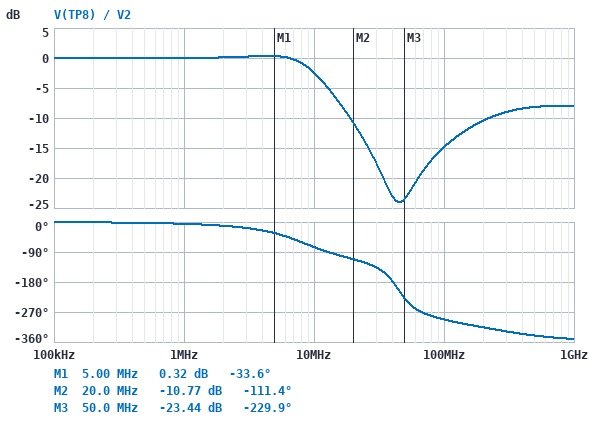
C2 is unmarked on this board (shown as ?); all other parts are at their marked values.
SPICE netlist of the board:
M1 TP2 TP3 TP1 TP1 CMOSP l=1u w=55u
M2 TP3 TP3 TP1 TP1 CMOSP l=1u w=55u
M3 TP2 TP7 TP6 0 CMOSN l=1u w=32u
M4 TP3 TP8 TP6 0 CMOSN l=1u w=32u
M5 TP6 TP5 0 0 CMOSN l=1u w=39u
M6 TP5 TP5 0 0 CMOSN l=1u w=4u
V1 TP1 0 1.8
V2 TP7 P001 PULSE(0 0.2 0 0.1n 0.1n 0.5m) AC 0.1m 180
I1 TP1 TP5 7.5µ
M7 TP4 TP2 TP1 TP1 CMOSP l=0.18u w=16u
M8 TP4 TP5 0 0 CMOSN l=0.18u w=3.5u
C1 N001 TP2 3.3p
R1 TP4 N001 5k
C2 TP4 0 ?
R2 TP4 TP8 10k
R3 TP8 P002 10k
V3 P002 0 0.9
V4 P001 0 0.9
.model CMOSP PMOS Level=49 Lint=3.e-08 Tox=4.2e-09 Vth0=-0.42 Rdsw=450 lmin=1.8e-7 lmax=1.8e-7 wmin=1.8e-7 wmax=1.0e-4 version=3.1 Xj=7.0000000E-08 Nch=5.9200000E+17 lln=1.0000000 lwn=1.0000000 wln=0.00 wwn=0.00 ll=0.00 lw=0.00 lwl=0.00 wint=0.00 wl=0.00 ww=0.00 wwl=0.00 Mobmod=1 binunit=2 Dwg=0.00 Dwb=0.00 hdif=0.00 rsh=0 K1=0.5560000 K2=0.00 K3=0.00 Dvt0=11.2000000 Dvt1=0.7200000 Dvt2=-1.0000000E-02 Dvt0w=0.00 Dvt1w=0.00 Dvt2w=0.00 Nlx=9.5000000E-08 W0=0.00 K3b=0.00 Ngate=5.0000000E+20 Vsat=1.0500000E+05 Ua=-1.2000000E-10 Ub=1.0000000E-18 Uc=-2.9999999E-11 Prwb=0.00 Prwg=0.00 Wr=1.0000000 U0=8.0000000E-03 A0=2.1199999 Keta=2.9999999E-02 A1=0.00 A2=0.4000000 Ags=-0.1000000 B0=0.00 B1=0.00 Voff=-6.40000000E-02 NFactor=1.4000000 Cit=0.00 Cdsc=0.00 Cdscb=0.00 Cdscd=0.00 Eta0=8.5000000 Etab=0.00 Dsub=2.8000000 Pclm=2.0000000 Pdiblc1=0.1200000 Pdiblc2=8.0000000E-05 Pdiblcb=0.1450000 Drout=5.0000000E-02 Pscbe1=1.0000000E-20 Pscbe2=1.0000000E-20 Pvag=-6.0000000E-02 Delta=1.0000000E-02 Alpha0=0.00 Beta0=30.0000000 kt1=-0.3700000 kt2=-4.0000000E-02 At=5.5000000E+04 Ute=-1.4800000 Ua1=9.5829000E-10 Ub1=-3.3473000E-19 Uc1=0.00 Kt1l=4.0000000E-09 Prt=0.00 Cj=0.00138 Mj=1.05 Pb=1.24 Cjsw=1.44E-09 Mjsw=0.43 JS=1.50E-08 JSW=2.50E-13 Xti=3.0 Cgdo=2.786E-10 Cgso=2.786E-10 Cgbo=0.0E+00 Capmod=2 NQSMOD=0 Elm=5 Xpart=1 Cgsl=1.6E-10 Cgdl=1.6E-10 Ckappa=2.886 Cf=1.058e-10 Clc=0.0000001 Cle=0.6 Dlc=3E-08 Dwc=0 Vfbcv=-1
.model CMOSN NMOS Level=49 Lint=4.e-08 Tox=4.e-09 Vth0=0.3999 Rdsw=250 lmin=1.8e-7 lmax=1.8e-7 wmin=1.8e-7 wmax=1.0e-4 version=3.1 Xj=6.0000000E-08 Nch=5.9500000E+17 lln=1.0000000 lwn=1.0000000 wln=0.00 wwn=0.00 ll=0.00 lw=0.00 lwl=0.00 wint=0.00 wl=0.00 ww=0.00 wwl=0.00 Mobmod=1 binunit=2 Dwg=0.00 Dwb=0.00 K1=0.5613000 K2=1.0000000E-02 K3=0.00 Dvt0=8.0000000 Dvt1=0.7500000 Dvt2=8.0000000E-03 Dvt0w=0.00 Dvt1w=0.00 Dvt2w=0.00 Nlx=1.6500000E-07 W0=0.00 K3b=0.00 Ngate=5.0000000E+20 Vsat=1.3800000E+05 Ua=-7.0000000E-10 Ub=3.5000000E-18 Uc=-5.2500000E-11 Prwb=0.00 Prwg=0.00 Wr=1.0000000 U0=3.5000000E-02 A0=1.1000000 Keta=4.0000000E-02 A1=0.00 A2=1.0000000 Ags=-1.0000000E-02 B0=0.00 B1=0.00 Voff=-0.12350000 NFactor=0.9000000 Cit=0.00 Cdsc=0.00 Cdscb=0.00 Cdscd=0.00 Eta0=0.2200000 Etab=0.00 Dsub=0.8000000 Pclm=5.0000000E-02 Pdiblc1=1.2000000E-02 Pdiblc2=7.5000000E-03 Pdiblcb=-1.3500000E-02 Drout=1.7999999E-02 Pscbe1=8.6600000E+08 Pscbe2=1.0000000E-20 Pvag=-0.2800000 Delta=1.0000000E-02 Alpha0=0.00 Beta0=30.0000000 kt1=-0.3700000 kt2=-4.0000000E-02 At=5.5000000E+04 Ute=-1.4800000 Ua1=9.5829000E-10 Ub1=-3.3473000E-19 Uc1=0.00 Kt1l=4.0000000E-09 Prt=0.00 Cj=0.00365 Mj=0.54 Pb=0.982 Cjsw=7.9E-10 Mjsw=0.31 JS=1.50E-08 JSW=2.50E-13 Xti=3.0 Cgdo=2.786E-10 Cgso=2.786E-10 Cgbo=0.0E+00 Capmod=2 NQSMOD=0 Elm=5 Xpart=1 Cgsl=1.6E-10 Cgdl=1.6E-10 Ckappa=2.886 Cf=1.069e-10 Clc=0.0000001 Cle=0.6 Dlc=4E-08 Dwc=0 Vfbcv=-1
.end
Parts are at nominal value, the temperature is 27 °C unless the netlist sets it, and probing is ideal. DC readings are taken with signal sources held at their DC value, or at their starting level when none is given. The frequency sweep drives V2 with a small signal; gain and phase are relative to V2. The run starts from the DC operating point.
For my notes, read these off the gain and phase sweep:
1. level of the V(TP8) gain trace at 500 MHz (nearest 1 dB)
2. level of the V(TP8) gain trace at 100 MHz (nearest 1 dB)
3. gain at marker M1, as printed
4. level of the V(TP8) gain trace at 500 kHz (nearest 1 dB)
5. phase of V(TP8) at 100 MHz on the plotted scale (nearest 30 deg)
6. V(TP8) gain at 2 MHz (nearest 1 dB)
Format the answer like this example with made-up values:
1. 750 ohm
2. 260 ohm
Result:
1. -8 dB
2. -15 dB
3. 0.32 dB
4. 0 dB
5. -300 deg
6. 0 dB
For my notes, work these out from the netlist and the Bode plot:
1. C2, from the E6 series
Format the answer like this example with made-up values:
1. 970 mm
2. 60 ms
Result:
1. 47 pF
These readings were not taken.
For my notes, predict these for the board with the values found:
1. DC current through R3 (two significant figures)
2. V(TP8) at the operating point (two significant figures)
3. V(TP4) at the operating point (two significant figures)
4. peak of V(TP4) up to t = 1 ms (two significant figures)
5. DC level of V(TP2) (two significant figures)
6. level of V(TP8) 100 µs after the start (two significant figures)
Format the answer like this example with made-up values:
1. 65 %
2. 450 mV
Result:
1. 310 nA
2. 900 mV
3. 910 mV
4. 1.3 V
5. 1.4 V
6. 1.1 V
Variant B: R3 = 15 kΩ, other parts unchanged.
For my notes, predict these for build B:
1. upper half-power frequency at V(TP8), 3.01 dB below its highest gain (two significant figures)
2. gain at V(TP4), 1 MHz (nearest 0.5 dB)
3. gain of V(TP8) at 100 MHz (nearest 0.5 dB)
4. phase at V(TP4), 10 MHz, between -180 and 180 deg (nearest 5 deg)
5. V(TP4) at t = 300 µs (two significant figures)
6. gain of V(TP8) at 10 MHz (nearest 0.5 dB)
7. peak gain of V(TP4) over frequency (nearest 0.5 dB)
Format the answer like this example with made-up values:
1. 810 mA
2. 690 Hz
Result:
1. 12 MHz
2. 4.5 dB
3. -13.5 dB
4. -65 deg
5. 1.2 V
6. -1.0 dB
7. 5.0 dB
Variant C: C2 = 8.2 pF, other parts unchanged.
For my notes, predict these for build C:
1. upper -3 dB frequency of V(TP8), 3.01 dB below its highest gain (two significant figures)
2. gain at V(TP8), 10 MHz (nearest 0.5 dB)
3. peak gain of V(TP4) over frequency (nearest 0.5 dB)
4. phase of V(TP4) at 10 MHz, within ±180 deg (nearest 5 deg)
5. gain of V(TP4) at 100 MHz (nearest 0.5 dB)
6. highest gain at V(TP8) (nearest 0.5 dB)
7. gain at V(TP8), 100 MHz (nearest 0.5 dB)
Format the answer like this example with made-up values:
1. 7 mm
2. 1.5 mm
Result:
1. 11 MHz
2. -3.0 dB
3. 6.0 dB
4. -30 deg
5. -7.0 dB
6. 0 dB
7. -17.0 dB
